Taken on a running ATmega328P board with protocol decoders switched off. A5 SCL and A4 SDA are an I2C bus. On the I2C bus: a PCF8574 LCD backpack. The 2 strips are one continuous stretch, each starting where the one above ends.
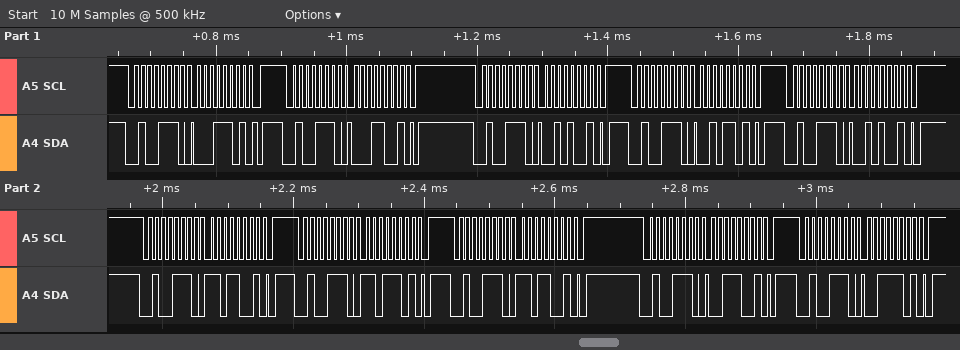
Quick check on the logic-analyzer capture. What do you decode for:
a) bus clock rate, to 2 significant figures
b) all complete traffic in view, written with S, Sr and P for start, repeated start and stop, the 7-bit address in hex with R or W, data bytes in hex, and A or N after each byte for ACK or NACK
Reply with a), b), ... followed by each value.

a) 100 kHz
b) S 27W A 1D A P S 27W A 19 A P S 27W A 29 A P S 27W A 2D A P S 27W A 29 A P S 27W A D9 A P S 27W A DD A P S 27W A D9 A P S 27W A 39 A P S 27W A 3D A P
